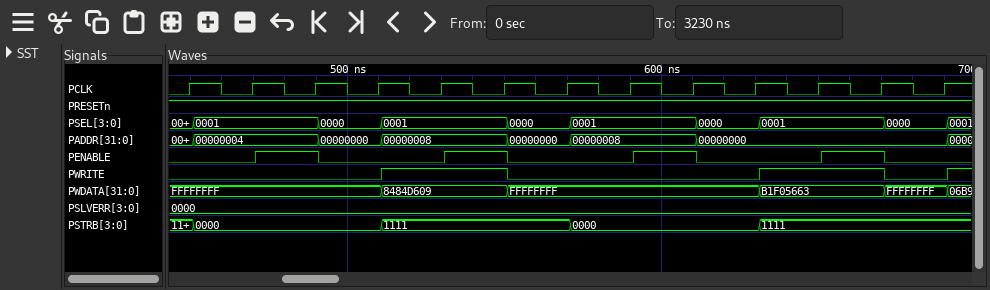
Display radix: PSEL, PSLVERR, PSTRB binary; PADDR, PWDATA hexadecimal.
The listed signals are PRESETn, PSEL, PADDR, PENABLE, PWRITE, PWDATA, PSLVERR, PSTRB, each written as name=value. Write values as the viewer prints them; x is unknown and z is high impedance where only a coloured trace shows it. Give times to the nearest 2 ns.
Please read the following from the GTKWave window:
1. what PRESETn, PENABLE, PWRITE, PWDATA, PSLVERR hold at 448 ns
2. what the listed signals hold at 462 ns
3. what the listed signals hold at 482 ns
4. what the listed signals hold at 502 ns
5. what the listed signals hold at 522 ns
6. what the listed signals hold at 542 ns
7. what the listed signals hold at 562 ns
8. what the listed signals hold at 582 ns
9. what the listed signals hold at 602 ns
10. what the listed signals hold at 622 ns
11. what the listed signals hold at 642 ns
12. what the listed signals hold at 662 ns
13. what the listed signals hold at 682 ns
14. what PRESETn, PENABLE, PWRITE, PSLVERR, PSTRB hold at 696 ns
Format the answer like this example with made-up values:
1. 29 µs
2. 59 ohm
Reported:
1. PRESETn=1, PENABLE=0, PWRITE=0, PWDATA=FFFFFFFF, PSLVERR=0000
2. PRESETn=1, PSEL=0001, PADDR=00000004, PENABLE=0, PWRITE=0, PWDATA=FFFFFFFF, PSLVERR=0000, PSTRB=0000
3. PRESETn=1, PSEL=0001, PADDR=00000004, PENABLE=1, PWRITE=0, PWDATA=FFFFFFFF, PSLVERR=0000, PSTRB=0000
4. PRESETn=1, PSEL=0000, PADDR=00000000, PENABLE=0, PWRITE=0, PWDATA=FFFFFFFF, PSLVERR=0000, PSTRB=0000
5. PRESETn=1, PSEL=0001, PADDR=00000008, PENABLE=0, PWRITE=1, PWDATA=8484D609, PSLVERR=0000, PSTRB=1111
6. PRESETn=1, PSEL=0001, PADDR=00000008, PENABLE=1, PWRITE=1, PWDATA=8484D609, PSLVERR=0000, PSTRB=1111
7. PRESETn=1, PSEL=0000, PADDR=00000000, PENABLE=0, PWRITE=0, PWDATA=FFFFFFFF, PSLVERR=0000, PSTRB=1111
8. PRESETn=1, PSEL=0001, PADDR=00000008, PENABLE=0, PWRITE=0, PWDATA=FFFFFFFF, PSLVERR=0000, PSTRB=0000
9. PRESETn=1, PSEL=0001, PADDR=00000008, PENABLE=1, PWRITE=0, PWDATA=FFFFFFFF, PSLVERR=0000, PSTRB=0000
10. PRESETn=1, PSEL=0000, PADDR=00000000, PENABLE=0, PWRITE=0, PWDATA=FFFFFFFF, PSLVERR=0000, PSTRB=0000
11. PRESETn=1, PSEL=0001, PADDR=00000000, PENABLE=0, PWRITE=1, PWDATA=B1F05663, PSLVERR=0000, PSTRB=1111
12. PRESETn=1, PSEL=0001, PADDR=00000000, PENABLE=1, PWRITE=1, PWDATA=B1F05663, PSLVERR=0000, PSTRB=1111
13. PRESETn=1, PSEL=0000, PADDR=00000000, PENABLE=0, PWRITE=0, PWDATA=FFFFFFFF, PSLVERR=0000, PSTRB=1111
14. PRESETn=1, PENABLE=0, PWRITE=1, PSLVERR=0000, PSTRB=1111
